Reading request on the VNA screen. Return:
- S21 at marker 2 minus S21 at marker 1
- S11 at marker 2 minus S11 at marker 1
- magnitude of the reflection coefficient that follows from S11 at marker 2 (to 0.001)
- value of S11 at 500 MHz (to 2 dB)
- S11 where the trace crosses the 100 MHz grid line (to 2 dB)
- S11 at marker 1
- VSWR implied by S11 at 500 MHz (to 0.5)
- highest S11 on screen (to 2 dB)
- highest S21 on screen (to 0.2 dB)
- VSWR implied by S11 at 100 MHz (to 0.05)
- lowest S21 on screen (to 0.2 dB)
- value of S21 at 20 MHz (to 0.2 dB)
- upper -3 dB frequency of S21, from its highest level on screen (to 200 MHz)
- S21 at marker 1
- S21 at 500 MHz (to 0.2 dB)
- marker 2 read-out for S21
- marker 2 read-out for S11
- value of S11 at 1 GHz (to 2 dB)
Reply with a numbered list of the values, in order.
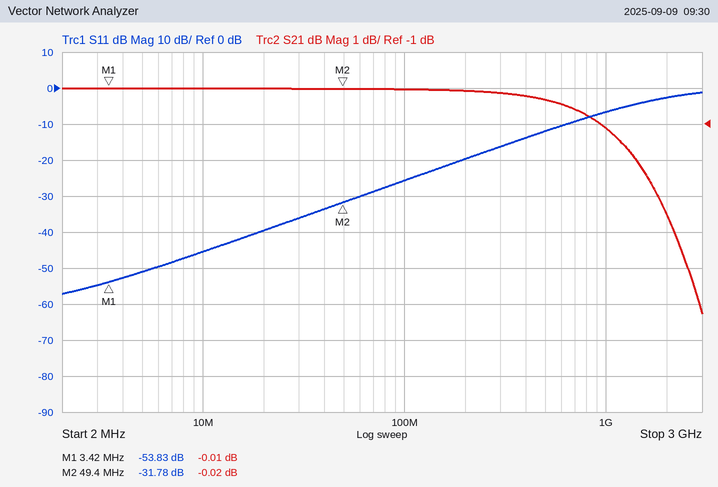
1. -0.01 dB
2. 22.05 dB
3. 0.026
4. -12 dB
5. -26 dB
6. -53.83 dB
7. 1.5
8. -2 dB
9. 0.0 dB
10. 1.10
11. -6.2 dB
12. 0.0 dB
13. 1.8 GHz
14. -0.01 dB
15. -0.4 dB
16. -0.02 dB
17. -31.78 dB
18. -6 dB
